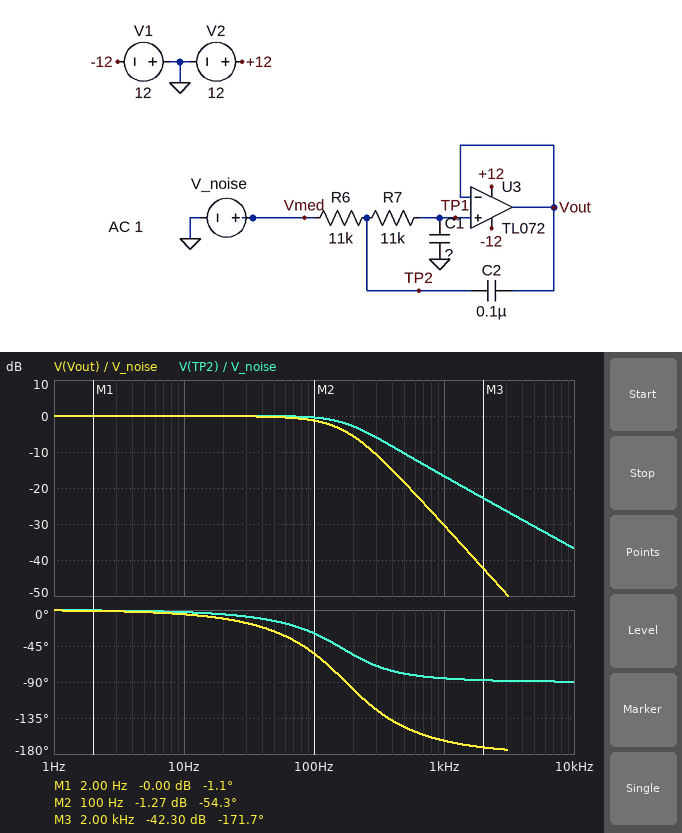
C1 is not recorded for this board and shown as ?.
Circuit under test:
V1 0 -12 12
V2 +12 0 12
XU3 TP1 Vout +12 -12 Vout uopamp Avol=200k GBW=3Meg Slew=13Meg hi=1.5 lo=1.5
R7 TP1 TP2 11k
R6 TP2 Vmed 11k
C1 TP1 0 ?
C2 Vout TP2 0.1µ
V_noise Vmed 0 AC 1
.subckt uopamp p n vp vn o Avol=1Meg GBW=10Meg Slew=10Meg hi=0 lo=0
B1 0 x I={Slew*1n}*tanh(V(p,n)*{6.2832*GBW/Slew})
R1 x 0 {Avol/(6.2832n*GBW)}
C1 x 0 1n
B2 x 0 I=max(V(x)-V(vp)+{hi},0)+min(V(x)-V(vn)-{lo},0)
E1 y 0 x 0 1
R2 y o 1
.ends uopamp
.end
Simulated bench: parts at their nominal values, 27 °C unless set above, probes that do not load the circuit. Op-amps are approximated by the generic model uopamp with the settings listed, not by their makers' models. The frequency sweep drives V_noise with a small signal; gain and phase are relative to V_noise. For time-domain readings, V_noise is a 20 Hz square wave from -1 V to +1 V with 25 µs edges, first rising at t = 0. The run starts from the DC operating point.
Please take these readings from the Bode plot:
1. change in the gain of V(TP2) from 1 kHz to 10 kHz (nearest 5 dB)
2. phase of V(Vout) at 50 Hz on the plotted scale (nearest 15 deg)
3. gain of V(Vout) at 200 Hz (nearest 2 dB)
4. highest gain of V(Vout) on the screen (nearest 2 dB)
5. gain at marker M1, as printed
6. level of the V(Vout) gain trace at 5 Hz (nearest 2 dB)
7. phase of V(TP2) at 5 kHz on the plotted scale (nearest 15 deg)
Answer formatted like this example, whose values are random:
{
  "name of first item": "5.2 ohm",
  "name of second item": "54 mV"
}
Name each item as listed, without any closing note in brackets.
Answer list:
{
  "change in the gain of V(TP2) from 1 kHz to 10 kHz": "-20 dB",
  "phase of V(Vout) at 50 Hz on the plotted scale": "-30 deg",
  "gain of V(Vout) at 200 Hz": "-6 dB",
  "highest gain of V(Vout) on the screen": "0 dB",
  "gain at marker M1, as printed": "-0.00 dB",
  "level of the V(Vout) gain trace at 5 Hz": "0 dB",
  "phase of V(TP2) at 5 kHz on the plotted scale": "-90 deg"
}
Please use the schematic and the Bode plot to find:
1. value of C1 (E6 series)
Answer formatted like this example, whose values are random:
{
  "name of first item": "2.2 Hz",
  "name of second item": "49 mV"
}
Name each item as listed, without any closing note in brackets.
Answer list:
{
  "value of C1": "68 nF"
}
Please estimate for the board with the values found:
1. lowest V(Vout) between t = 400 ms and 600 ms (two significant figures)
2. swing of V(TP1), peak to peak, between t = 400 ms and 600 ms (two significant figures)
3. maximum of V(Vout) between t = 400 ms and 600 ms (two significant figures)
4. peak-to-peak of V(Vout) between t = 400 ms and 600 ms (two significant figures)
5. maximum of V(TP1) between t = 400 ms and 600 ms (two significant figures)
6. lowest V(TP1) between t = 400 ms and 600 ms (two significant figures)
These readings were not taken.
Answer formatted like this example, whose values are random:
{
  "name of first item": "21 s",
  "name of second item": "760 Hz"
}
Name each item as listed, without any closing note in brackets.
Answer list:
{
  "lowest V(Vout) between t = 400 ms and 600 ms": "-1.0 V",
  "swing of V(TP1), peak to peak, between t = 400 ms and 600 ms": "2.0 V",
  "maximum of V(Vout) between t = 400 ms and 600 ms": "1.0 V",
  "peak-to-peak of V(Vout) between t = 400 ms and 600 ms": "2.0 V",
  "maximum of V(TP1) between t = 400 ms and 600 ms": "1.0 V",
  "lowest V(TP1) between t = 400 ms and 600 ms": "-1.0 V"
}
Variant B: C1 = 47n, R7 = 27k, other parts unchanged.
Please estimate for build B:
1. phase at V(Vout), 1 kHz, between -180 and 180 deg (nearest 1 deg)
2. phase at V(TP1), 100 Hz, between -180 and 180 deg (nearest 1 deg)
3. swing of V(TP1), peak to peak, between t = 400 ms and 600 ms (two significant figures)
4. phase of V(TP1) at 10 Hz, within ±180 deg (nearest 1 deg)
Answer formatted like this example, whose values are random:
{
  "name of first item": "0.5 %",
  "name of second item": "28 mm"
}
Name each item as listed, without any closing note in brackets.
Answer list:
{
  "phase at V(Vout), 1 kHz, between -180 and 180 deg": "-168 deg",
  "phase at V(TP1), 100 Hz, between -180 and 180 deg": "-68 deg",
  "swing of V(TP1), peak to peak, between t = 400 ms and 600 ms": "2.1 V",
  "phase of V(TP1) at 10 Hz, within ±180 deg": "-6 deg"
}
